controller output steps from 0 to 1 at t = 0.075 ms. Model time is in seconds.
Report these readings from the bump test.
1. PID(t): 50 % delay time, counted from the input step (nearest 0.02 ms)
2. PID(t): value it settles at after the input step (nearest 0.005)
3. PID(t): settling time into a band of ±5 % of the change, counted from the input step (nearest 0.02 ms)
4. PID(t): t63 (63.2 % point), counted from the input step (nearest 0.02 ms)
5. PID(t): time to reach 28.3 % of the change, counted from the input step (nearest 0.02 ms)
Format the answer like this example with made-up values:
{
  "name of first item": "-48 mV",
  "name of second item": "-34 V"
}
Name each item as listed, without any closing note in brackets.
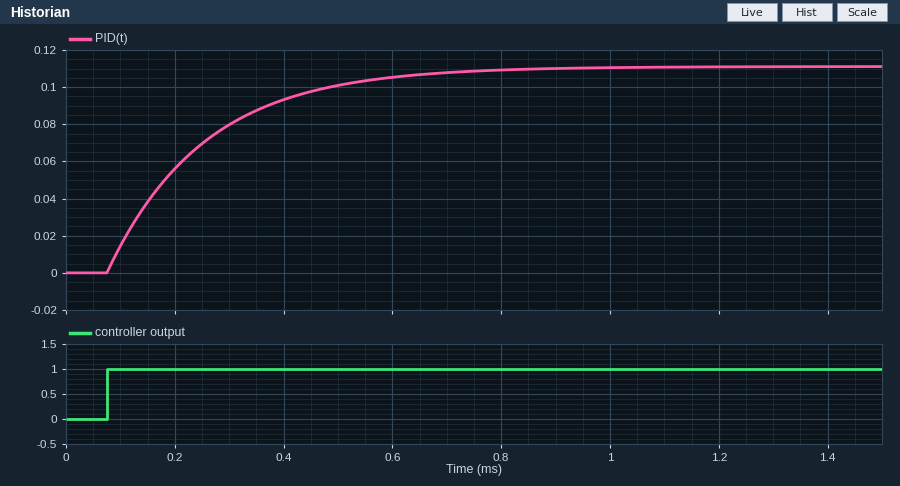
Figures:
{
  "PID(t): 50 % delay time, counted from the input step": "0.12 ms",
  "PID(t): value it settles at after the input step": "0.110",
  "PID(t): settling time into a band of ±5 % of the change, counted from the input step": "0.54 ms",
  "PID(t): t63 (63.2 % point), counted from the input step": "0.18 ms",
  "PID(t): time to reach 28.3 % of the change, counted from the input step": "0.06 ms"
}
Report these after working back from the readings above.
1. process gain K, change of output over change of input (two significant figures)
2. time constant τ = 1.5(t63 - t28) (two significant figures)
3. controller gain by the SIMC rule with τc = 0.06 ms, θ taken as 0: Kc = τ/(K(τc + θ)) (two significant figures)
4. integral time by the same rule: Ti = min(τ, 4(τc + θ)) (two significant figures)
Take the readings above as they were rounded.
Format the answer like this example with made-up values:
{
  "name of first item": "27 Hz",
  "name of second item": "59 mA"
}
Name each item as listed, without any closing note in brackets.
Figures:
{
  "process gain K, change of output over change of input": "0.11",
  "time constant τ = 1.5(t63 - t28)": "0.18 ms",
  "controller gain by the SIMC rule with τc = 0.06 ms, θ taken as 0: Kc = τ/(K(τc + θ))": "27",
  "integral time by the same rule: Ti = min(τ, 4(τc + θ))": "0.18 ms"
}
